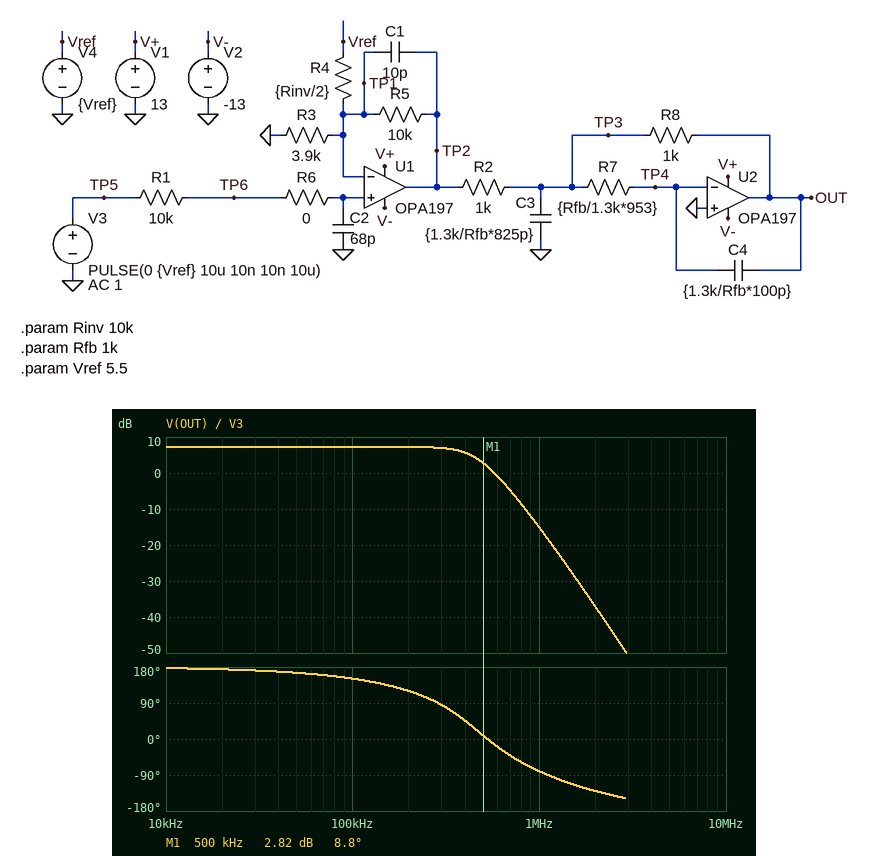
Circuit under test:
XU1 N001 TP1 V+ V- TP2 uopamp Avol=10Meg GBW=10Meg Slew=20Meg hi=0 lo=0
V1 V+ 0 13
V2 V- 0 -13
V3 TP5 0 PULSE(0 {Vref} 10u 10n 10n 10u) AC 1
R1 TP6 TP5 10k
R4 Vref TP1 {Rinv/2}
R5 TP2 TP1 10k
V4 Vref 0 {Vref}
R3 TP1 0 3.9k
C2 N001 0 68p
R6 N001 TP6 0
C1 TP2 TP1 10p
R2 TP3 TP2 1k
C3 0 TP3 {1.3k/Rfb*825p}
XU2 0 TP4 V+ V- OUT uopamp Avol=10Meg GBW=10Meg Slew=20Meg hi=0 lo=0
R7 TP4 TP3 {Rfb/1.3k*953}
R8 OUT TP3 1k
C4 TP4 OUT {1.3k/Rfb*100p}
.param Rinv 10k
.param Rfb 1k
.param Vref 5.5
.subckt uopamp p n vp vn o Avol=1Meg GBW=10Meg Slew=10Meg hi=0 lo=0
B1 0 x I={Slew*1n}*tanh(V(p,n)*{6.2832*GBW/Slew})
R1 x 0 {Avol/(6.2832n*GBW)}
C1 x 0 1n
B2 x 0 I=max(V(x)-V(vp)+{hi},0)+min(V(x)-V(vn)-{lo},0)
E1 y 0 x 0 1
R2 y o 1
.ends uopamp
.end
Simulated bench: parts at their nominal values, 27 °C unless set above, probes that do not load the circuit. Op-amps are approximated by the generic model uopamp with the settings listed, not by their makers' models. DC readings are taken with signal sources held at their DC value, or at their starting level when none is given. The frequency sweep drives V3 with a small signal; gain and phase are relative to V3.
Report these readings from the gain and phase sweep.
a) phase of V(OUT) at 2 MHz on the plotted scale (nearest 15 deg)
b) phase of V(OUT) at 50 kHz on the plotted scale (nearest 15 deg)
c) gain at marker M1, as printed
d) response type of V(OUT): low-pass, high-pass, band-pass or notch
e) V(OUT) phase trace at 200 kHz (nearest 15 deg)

-135 deg
165 deg
2.82 dB
low-pass
120 deg
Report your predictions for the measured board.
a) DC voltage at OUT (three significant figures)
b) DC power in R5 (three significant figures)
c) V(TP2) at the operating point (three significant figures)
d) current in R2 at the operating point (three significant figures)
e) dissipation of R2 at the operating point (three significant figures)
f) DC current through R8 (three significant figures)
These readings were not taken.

11.0 V
12.1 mW
-11.0 V
11.0 mA
121 mW
11.0 mA
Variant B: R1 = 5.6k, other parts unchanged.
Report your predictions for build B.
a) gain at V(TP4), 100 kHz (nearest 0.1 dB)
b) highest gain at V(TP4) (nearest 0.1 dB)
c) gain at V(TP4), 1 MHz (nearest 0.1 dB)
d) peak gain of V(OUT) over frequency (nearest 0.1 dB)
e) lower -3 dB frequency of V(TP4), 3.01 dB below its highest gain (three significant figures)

-27.8 dB
-17.2 dB
-30.1 dB
12.2 dB
238 kHz
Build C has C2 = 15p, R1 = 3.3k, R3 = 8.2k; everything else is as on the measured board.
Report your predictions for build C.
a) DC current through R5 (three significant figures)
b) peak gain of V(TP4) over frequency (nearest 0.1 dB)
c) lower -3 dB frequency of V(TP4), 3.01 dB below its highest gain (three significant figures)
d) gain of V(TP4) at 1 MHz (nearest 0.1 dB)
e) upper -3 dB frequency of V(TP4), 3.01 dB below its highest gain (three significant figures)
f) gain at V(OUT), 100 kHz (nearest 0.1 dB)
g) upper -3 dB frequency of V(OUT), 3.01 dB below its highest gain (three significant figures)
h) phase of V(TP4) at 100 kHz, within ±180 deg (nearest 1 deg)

1.10 mA
-13.1 dB
271 kHz
-21.8 dB
669 kHz
14.5 dB
512 kHz
70 deg
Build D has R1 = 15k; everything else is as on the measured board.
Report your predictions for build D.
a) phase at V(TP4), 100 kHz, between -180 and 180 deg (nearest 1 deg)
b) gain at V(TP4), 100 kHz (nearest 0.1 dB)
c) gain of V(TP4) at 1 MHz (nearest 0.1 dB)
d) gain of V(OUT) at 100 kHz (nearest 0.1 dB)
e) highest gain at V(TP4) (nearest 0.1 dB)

61 deg
-36.3 dB
-38.7 dB
3.7 dB
-25.8 dB
